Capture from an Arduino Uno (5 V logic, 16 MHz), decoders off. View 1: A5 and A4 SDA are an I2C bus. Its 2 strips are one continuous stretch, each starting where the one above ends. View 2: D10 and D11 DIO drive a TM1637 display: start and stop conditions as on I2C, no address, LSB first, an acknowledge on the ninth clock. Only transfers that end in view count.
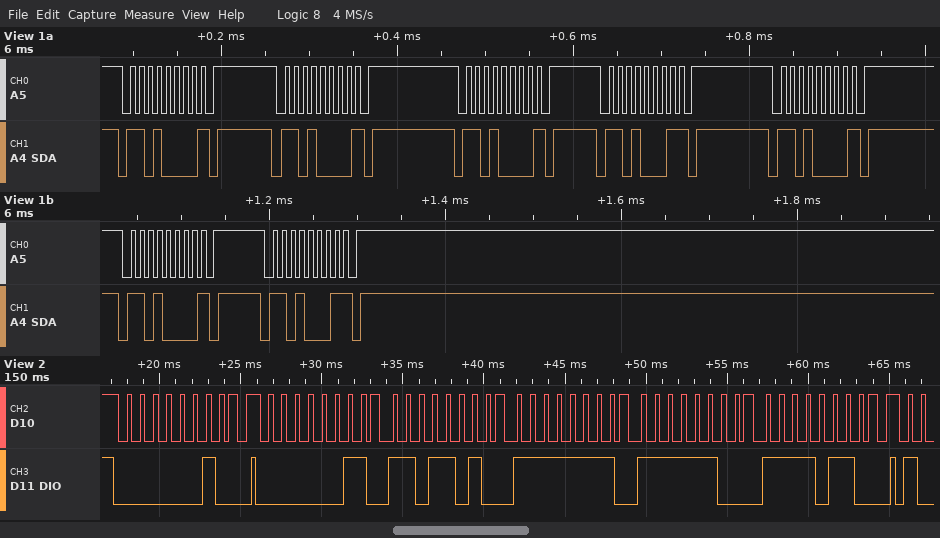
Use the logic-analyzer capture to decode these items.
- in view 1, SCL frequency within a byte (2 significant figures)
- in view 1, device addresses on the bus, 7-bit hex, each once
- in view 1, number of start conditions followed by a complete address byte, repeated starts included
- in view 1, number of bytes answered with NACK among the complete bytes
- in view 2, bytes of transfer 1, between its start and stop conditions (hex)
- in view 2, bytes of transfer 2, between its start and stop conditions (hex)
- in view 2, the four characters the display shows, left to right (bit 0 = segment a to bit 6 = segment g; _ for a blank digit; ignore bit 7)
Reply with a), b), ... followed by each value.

a) 100 kHz
b) 0x68
c) 7
d) 7
e) 40
f) C0 5B FF 3F 6F
g) 2809
